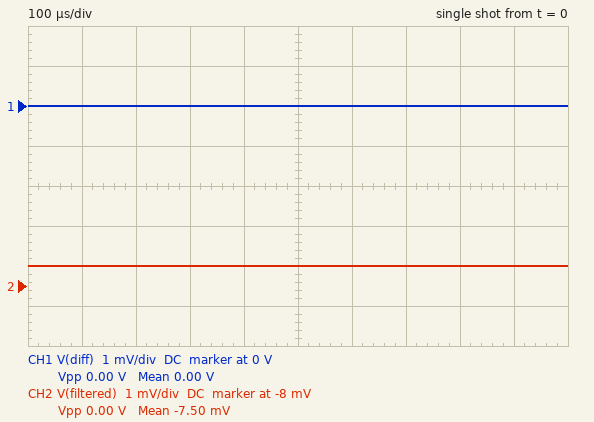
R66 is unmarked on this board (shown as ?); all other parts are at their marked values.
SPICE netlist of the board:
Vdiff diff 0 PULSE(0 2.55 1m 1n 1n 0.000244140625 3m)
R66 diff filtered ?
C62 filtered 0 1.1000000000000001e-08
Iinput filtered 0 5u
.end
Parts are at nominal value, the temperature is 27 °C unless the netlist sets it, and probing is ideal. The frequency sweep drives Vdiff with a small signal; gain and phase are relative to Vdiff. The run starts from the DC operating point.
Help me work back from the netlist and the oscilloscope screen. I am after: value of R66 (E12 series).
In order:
1.5 kΩ
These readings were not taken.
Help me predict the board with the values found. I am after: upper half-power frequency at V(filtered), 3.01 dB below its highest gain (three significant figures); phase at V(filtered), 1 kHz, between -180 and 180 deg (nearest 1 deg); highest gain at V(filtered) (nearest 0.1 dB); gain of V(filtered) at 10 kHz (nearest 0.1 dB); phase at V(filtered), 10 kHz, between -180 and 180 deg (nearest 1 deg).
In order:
9.65 kHz
-6 deg
0 dB
-3.2 dB
-46 deg
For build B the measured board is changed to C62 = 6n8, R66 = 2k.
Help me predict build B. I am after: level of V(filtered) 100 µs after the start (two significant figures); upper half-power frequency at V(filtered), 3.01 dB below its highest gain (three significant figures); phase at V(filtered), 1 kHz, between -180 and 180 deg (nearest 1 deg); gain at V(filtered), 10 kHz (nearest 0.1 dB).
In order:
-10 mV
11.7 kHz
-5 deg
-2.4 dB
